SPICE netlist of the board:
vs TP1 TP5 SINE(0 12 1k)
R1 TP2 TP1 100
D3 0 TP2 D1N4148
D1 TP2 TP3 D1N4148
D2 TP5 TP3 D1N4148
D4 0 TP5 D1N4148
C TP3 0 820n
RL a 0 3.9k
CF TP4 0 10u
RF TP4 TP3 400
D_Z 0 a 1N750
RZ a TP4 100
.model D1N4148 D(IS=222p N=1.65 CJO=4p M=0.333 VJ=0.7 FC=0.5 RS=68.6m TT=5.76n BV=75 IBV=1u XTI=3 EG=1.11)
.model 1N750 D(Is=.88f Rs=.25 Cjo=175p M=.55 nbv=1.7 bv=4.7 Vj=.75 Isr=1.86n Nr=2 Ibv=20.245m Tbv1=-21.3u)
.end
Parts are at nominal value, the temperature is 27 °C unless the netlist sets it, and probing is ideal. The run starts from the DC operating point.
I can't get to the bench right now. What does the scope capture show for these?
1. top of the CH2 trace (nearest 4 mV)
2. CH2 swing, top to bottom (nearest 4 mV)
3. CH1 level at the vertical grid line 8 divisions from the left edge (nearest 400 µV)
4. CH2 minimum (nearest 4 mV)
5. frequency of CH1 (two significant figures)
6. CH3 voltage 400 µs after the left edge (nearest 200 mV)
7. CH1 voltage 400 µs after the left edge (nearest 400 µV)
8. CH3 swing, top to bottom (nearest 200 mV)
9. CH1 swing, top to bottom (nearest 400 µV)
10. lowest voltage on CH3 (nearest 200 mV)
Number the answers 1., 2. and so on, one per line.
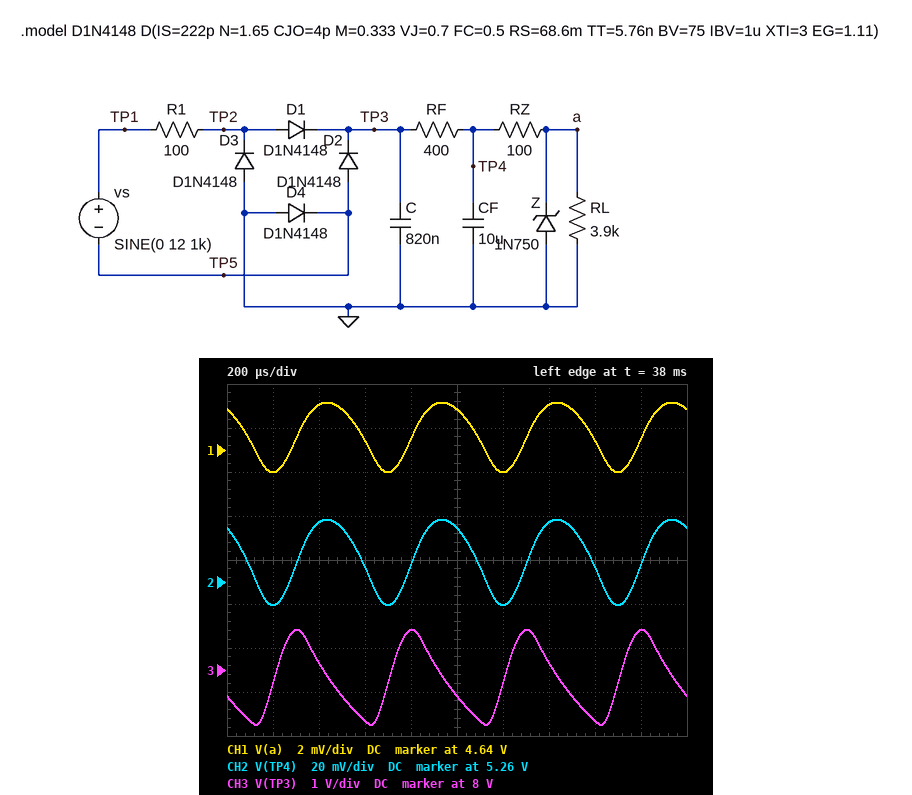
1. 5.288 V
2. 40 mV
3. 4.6404 V
4. 5.248 V
5. 2.0 kHz
6. 8.2 V
7. 4.6420 V
8. 2.2 V
9. 3.2 mV
10. 6.8 V
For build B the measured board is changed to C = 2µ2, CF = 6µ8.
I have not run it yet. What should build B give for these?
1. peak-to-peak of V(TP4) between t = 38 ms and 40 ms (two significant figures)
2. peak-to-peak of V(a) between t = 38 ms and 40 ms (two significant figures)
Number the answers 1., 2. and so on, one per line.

1. 23 mV
2. 1.8 mV
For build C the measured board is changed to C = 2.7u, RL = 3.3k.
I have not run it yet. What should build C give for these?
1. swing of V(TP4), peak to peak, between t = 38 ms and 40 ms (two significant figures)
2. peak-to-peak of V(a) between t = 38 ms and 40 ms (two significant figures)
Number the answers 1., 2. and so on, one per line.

1. 13 mV
2. 1.0 mV
